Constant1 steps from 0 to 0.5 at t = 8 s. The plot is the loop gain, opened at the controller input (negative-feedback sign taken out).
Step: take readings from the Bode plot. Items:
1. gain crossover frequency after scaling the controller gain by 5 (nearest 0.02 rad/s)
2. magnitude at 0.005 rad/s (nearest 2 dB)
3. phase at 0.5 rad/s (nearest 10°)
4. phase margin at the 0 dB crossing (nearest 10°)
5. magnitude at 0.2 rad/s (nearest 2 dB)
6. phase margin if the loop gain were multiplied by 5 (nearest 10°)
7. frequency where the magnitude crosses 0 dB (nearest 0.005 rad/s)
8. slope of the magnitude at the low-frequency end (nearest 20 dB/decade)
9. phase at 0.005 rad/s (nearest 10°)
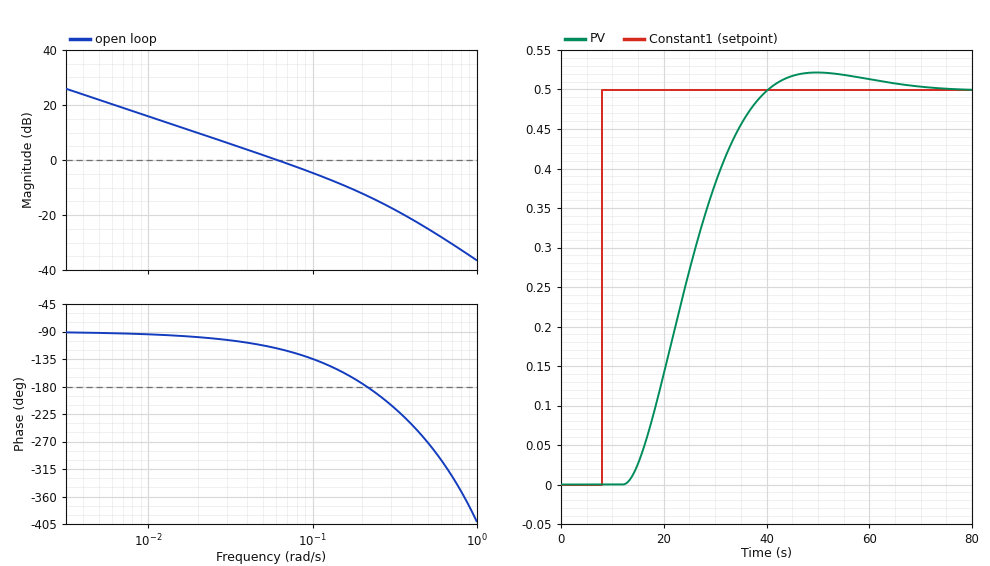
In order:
0.24 rad/s
22 dB
-270°
60°
-12 dB
-10°
0.060 rad/s
-20 dB/decade
-90°
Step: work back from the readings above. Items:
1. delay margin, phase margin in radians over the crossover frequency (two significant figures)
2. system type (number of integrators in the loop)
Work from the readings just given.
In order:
17 s
1
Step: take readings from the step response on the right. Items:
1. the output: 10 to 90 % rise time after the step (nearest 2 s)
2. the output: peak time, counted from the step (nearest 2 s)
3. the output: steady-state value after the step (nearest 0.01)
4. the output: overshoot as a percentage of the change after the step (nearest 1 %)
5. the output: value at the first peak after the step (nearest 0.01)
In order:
18 s
42 s
0.50
4 %
0.52
